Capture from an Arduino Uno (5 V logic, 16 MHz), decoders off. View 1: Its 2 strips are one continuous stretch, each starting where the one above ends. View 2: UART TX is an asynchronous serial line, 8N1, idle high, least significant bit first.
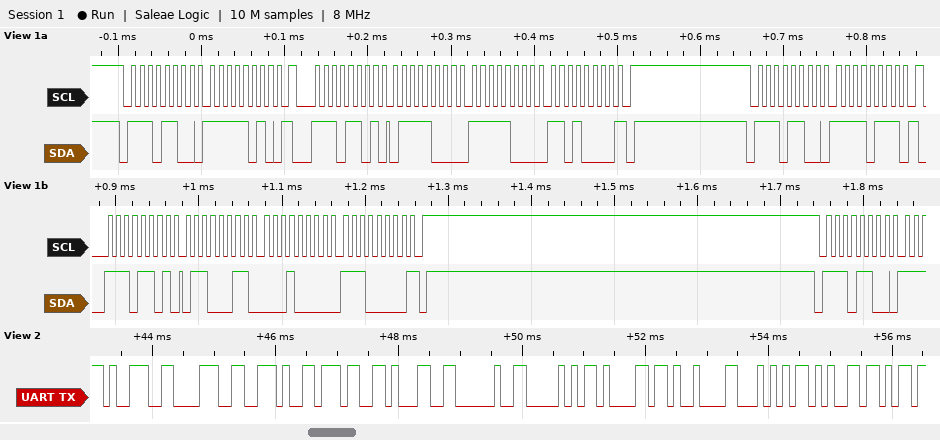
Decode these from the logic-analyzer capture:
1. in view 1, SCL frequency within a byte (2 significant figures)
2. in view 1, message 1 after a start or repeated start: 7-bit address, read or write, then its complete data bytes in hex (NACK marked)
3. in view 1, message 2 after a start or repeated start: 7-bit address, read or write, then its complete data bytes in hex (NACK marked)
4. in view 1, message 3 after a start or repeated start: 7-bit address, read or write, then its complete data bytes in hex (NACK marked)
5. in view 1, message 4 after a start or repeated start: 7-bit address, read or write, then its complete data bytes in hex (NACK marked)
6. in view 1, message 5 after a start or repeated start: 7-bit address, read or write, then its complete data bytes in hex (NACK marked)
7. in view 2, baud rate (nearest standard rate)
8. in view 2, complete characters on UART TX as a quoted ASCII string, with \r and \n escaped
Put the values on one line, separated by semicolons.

100 kHz; 0x76 write: FA; 0x76 read: 78 F8 D0 NACK; 0x76 write: F7; 0x76 read: 63 10 E0 NACK; 0x76 write; 9600 baud; "98.71 Pa\tTe"
